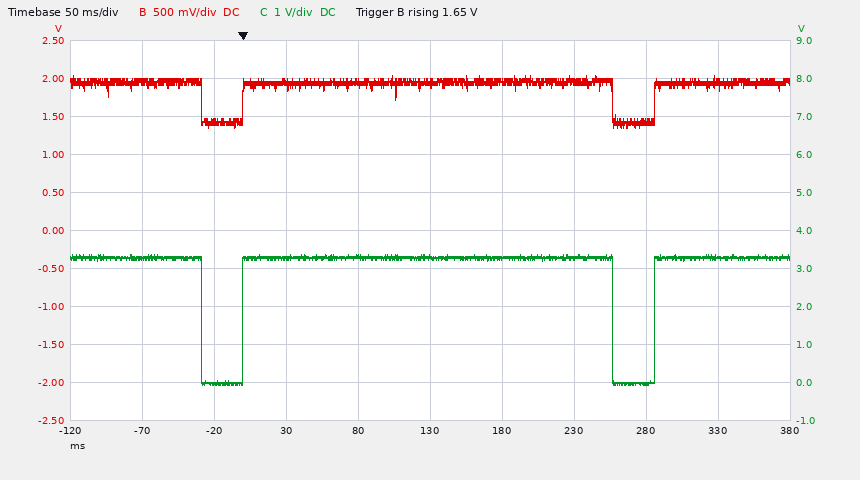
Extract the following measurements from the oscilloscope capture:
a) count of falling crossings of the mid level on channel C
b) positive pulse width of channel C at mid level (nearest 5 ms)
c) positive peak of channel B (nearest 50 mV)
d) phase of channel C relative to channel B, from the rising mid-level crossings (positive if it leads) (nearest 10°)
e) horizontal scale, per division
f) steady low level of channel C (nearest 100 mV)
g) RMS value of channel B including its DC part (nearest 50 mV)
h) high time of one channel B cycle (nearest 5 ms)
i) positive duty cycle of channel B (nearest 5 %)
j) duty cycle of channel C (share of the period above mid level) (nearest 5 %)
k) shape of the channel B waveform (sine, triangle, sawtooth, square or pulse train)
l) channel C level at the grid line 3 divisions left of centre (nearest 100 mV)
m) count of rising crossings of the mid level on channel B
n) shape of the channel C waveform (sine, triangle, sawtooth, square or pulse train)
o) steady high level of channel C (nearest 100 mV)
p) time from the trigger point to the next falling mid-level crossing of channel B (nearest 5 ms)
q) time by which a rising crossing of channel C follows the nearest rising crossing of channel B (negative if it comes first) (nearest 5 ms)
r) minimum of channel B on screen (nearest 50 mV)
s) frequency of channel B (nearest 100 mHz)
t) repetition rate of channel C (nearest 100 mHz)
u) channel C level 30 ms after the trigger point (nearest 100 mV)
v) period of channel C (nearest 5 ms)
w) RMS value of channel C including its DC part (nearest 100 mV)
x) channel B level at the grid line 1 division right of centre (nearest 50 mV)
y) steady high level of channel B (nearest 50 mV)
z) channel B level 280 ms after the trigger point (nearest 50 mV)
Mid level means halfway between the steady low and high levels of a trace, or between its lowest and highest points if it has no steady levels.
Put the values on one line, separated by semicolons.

2; 255 ms; 2.05 V; 0°; 50 ms; 0.0 V; 1.90 V; 255 ms; 90 %; 90 %; pulse train; 0.0 V; 2; pulse train; 3.3 V; 255 ms; 0 ms; 1.35 V; 3.5 Hz; 3.5 Hz; 3.3 V; 285 ms; 3.1 V; 1.95 V; 1.95 V; 1.45 V
